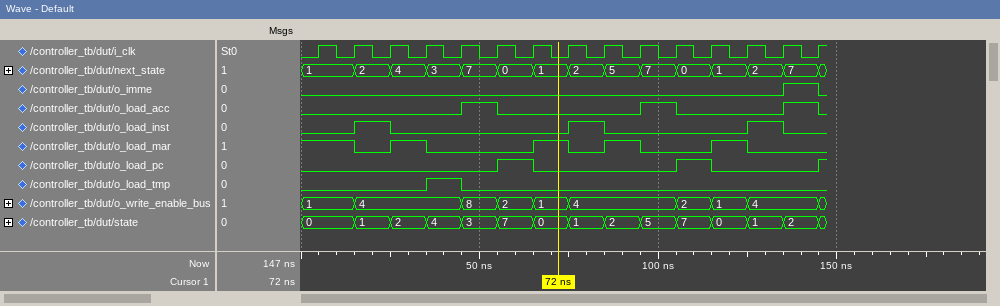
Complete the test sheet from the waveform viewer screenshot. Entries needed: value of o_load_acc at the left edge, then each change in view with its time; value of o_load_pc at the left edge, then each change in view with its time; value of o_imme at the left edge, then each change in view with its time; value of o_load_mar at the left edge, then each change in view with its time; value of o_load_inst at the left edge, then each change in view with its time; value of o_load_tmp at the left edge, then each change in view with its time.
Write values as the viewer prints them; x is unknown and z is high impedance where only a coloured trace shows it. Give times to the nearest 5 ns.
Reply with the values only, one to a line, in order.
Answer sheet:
0, 1 at 45 ns, 0 at 55 ns, 1 at 95 ns, 0 at 105 ns, 1 at 135 ns, 0 at 145 ns
0, 1 at 55 ns, 0 at 65 ns, 1 at 105 ns, 0 at 115 ns, 1 at 145 ns
0, 1 at 135 ns, 0 at 145 ns
1, 0 at 15 ns, 1 at 25 ns, 0 at 35 ns, 1 at 65 ns, 0 at 75 ns, 1 at 85 ns, 0 at 95 ns, 1 at 115 ns, 0 at 125 ns
0, 1 at 15 ns, 0 at 25 ns, 1 at 75 ns, 0 at 85 ns, 1 at 125 ns, 0 at 135 ns
0, 1 at 35 ns, 0 at 45 ns
